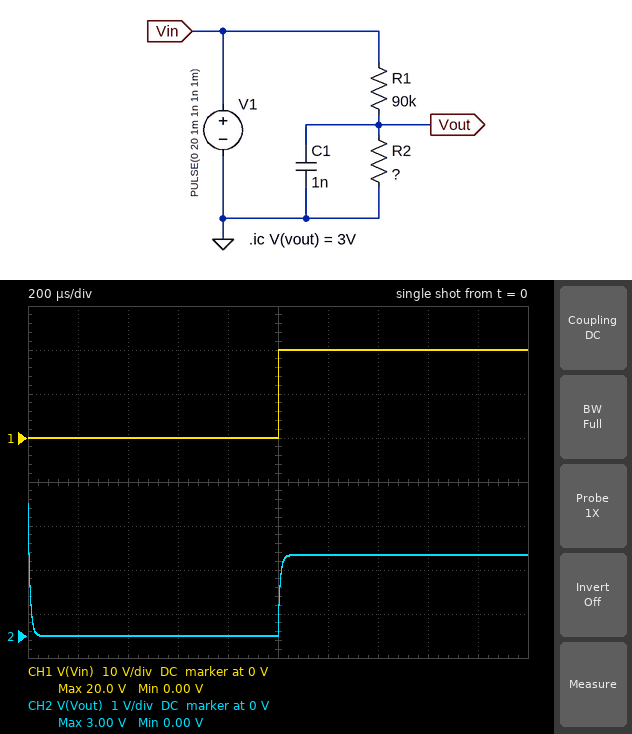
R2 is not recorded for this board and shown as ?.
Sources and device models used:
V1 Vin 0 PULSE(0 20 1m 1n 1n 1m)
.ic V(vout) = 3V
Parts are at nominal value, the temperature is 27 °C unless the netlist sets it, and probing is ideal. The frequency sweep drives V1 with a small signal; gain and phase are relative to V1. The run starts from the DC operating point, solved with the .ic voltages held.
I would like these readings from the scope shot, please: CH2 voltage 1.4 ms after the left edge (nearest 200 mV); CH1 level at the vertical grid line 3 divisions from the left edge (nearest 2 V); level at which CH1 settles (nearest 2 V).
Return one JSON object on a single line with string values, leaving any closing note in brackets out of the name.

{"CH2 voltage 1.4 ms after the left edge": "1.8 V", "CH1 level at the vertical grid line 3 divisions from the left edge": "0 V", "level at which CH1 settles": "20 V"}
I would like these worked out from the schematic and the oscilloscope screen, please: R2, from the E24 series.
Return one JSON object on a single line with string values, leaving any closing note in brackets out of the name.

{"R2, from the E24 series": "9.1 kΩ"}
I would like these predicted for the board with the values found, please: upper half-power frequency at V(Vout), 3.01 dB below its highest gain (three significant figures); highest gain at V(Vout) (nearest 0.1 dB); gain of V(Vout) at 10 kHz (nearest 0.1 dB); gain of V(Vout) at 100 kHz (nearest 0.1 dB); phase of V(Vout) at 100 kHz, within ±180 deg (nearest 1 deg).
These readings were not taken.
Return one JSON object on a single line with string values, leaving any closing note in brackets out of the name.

{"upper half-power frequency at V(Vout), 3.01 dB below its highest gain": "19.3 kHz", "highest gain at V(Vout)": "-20.7 dB", "gain of V(Vout) at 10 kHz": "-21.8 dB", "gain of V(Vout) at 100 kHz": "-35.2 dB", "phase of V(Vout) at 100 kHz, within ±180 deg": "-79 deg"}
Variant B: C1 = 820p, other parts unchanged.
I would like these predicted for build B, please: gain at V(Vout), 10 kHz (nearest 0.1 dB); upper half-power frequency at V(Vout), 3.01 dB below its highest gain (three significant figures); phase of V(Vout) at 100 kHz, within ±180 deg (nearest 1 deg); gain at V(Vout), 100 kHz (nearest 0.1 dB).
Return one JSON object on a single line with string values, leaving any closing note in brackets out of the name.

{"gain at V(Vout), 10 kHz": "-21.5 dB", "upper half-power frequency at V(Vout), 3.01 dB below its highest gain": "23.5 kHz", "phase of V(Vout) at 100 kHz, within ±180 deg": "-77 deg", "gain at V(Vout), 100 kHz": "-33.6 dB"}
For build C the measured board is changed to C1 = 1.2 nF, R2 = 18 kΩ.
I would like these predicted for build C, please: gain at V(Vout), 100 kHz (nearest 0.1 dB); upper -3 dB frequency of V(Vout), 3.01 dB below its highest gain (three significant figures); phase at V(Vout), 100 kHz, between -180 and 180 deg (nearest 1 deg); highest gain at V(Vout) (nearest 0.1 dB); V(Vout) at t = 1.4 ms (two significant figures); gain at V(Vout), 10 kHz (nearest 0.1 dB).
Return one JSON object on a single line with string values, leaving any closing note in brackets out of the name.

{"gain at V(Vout), 100 kHz": "-36.7 dB", "upper -3 dB frequency of V(Vout), 3.01 dB below its highest gain": "8.84 kHz", "phase at V(Vout), 100 kHz, between -180 and 180 deg": "-85 deg", "highest gain at V(Vout)": "-15.6 dB", "V(Vout) at t = 1.4 ms": "3.3 V", "gain at V(Vout), 10 kHz": "-19.1 dB"}
